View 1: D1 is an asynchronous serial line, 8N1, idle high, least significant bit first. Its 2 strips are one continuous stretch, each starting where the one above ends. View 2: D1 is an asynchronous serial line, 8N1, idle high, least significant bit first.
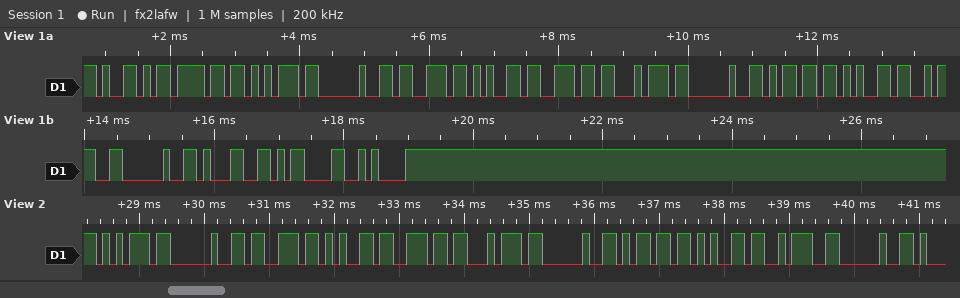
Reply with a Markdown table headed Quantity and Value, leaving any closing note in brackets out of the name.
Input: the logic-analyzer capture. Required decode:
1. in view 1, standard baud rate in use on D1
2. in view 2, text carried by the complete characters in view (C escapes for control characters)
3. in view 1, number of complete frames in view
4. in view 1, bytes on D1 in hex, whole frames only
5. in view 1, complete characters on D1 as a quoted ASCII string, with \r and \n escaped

| Quantity | Value |
|---|---|
| in view 1, standard baud rate in use on D1 | 9600 baud |
| in view 2, text carried by the complete characters in view | "u sent me: " |
| in view 1, number of complete frames in view | 16 |
| in view 1, bytes on D1 in hex, whole frames only | 59 6F 75 20 73 65 6E 74 20 6D 65 3A 20 31 0D 0A |
| in view 1, complete characters on D1 as a quoted ASCII string, with \r and \n escaped | "You sent me: 1\r\n" |
